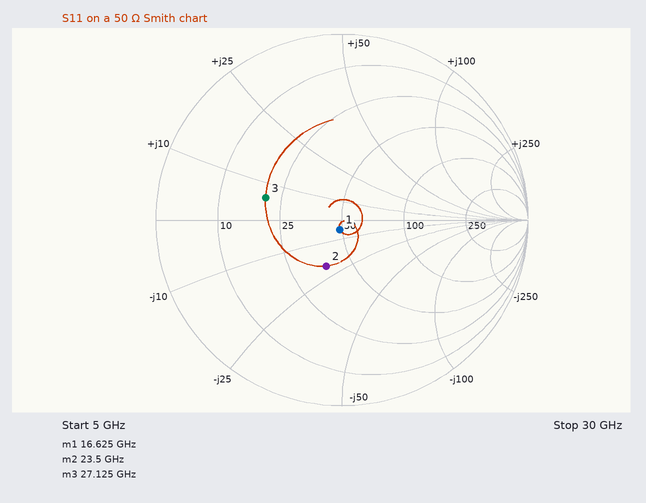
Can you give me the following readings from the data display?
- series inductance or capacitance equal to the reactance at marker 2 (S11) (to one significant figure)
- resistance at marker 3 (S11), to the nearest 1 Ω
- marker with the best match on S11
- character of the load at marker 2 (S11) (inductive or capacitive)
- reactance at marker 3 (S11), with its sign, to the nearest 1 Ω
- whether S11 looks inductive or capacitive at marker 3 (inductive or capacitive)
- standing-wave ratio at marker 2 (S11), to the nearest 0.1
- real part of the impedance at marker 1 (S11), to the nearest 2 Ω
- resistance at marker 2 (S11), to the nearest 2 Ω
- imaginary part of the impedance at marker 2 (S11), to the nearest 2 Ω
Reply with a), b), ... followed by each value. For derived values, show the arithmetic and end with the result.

a) C = 1/(2π × 23.5 GHz × 20 Ω) ≈ 339 fF, so 300 fF to one significant figure
b) 20 Ω
c) marker 1
d) capacitive
e) +6 Ω
f) inductive
g) 1.7
h) 48 Ω
i) 38 Ω
j) -20 Ω
